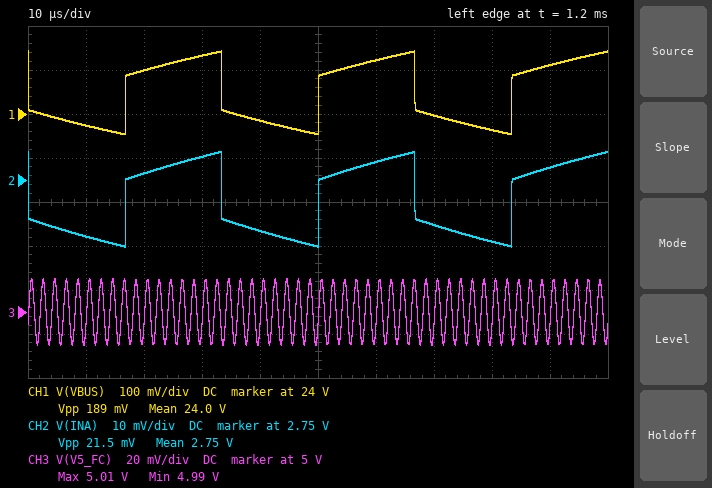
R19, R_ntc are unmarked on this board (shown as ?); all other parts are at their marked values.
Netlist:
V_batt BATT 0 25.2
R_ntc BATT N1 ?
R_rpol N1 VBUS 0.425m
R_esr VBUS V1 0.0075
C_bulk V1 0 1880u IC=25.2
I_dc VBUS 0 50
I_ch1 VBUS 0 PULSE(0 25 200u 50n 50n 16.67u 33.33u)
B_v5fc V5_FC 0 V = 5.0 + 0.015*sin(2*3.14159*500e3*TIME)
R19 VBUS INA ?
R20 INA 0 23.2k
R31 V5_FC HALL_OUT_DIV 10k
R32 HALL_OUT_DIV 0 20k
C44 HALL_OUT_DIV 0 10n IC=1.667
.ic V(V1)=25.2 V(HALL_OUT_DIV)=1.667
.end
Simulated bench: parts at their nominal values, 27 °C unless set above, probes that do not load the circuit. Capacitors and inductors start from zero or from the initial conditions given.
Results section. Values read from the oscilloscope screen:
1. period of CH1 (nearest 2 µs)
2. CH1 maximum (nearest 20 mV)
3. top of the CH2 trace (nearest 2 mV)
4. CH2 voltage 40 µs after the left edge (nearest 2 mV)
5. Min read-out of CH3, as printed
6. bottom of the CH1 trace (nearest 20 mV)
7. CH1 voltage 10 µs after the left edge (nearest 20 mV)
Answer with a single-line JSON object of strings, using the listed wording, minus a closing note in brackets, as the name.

{"period of CH1": "34 µs", "CH1 maximum": "24.14 V", "top of the CH2 trace": "2.756 V", "CH2 voltage 40 µs after the left edge": "2.738 V", "Min read-out of CH3, as printed": "4.99 V", "bottom of the CH1 trace": "23.96 V", "CH1 voltage 10 µs after the left edge": "23.98 V"}
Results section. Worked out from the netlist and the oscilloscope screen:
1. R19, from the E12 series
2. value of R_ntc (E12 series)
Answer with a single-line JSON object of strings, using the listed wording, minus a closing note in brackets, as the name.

{"R19, from the E12 series": "180 kΩ", "value of R_ntc": "0.018 Ω"}
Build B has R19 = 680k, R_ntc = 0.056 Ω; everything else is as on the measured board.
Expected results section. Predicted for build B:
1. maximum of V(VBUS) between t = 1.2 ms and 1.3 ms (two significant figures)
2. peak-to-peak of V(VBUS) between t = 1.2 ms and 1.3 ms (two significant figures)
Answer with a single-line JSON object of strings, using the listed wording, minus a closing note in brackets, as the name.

{"maximum of V(VBUS) between t = 1.2 ms and 1.3 ms": "22 V", "peak-to-peak of V(VBUS) between t = 1.2 ms and 1.3 ms": "250 mV"}
